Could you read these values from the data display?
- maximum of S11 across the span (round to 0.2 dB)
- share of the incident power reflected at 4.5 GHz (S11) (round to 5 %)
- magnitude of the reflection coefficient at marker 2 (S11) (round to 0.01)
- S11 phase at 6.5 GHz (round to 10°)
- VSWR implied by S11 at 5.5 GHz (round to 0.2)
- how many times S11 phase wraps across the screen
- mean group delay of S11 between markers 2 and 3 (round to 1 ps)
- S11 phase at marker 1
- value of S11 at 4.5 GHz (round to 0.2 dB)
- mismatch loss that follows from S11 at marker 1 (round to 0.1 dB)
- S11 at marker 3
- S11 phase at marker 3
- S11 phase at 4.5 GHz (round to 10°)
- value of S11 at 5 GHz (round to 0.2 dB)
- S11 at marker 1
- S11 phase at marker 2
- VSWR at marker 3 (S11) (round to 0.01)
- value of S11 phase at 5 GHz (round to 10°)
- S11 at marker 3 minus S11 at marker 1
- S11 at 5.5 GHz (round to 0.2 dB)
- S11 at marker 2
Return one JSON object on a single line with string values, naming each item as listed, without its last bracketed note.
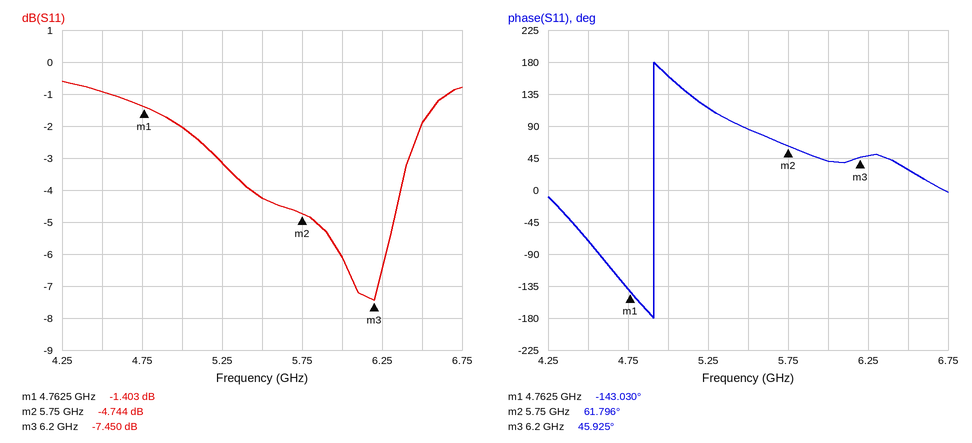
{"maximum of S11 across the span": "-0.6 dB", "share of the incident power reflected at 4.5 GHz (S11)": "80 %", "magnitude of the reflection coefficient at marker 2 (S11)": "0.58", "S11 phase at 6.5 GHz": "30°", "VSWR implied by S11 at 5.5 GHz": "4.2", "how many times S11 phase wraps across the screen": "1", "mean group delay of S11 between markers 2 and 3": "98 ps", "S11 phase at marker 1": "-143.030°", "value of S11 at 4.5 GHz": "-1.0 dB", "mismatch loss that follows from S11 at marker 1": "5.6 dB", "S11 at marker 3": "-7.450 dB", "S11 phase at marker 3": "45.925°", "S11 phase at 4.5 GHz": "-70°", "value of S11 at 5 GHz": "-2.0 dB", "S11 at marker 1": "-1.403 dB", "S11 phase at marker 2": "61.796°", "VSWR at marker 3 (S11)": "2.47", "value of S11 phase at 5 GHz": "160°", "S11 at marker 3 minus S11 at marker 1": "-6.047 dB", "S11 at 5.5 GHz": "-4.2 dB", "S11 at marker 2": "-4.744 dB"}
